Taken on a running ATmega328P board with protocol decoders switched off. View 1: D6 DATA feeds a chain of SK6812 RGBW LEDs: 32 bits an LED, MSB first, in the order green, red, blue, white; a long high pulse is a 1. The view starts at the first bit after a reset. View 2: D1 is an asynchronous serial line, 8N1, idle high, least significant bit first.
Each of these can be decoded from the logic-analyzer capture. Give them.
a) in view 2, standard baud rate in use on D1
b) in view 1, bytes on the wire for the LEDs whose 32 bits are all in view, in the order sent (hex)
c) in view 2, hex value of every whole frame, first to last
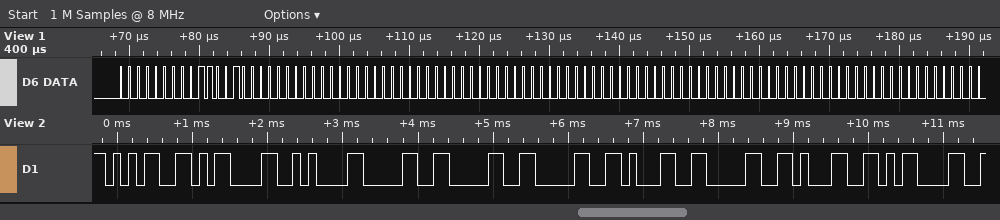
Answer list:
9600 baud
00 64 00 00 00 00 00 00 00 00 00 00
35 0D 0A 30 30 30 31 30 31 0D
